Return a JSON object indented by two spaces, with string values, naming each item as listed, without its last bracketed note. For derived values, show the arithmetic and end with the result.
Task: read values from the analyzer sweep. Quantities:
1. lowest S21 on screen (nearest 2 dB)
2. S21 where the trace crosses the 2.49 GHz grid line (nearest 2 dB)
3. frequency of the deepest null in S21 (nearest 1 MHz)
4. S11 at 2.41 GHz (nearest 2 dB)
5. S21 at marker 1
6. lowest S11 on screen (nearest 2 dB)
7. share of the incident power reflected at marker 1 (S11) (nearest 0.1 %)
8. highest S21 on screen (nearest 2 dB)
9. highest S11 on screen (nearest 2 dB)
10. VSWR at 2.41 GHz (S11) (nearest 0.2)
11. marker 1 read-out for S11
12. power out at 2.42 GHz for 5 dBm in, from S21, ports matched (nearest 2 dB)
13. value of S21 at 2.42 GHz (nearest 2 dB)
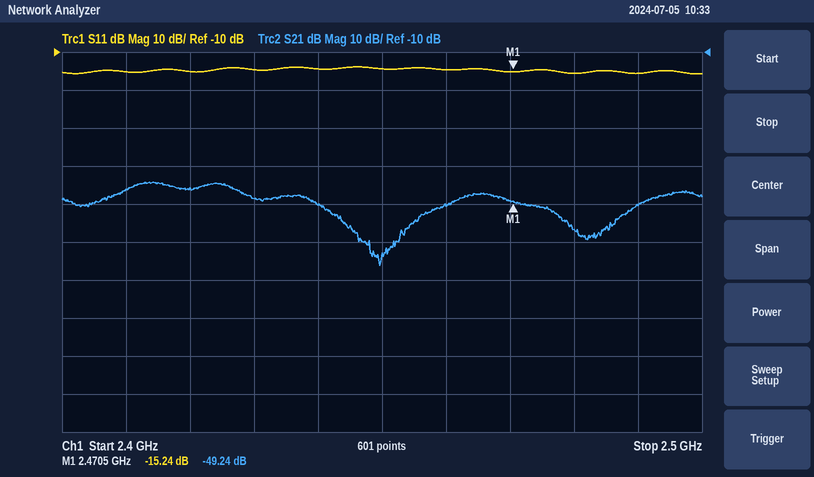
{
  "lowest S21 on screen": "-66 dB",
  "S21 where the trace crosses the 2.49 GHz grid line": "-50 dB",
  "frequency of the deepest null in S21": "2.450 GHz",
  "S11 at 2.41 GHz": "-16 dB",
  "S21 at marker 1": "-49.24 dB",
  "lowest S11 on screen": "-16 dB",
  "share of the incident power reflected at marker 1 (S11)": "10^(-15.24/10) ≈ 3.0 %",
  "highest S21 on screen": "-44 dB",
  "highest S11 on screen": "-14 dB",
  "VSWR at 2.41 GHz (S11)": "|Γ| = 10^(-16/20) = 0.1585; VSWR = (1 + 0.1585)/(1 − 0.1585) ≈ 1.4",
  "marker 1 read-out for S11": "-15.24 dB",
  "power out at 2.42 GHz for 5 dBm in, from S21, ports matched": "5 dBm + (-46 dB) = -40 dBm",
  "value of S21 at 2.42 GHz": "-46 dB"
}
